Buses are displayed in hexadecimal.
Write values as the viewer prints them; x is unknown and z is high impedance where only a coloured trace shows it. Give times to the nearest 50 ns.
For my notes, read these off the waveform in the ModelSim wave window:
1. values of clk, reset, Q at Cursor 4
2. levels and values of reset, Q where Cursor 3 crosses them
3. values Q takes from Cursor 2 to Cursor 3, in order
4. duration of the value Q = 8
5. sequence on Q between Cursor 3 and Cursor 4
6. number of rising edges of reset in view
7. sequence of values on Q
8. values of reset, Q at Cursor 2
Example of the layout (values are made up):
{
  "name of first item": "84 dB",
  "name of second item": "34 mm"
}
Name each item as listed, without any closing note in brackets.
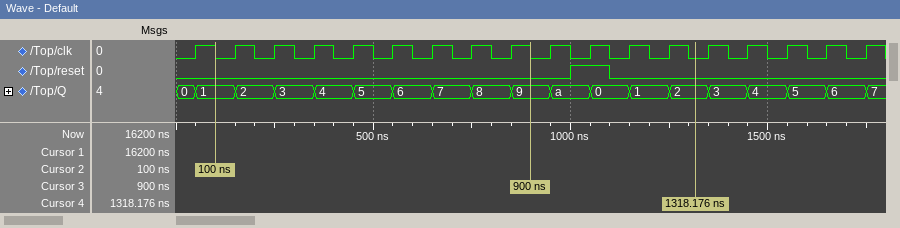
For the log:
{
  "values of clk, reset, Q at Cursor 4": "clk=0, reset=0, Q=2",
  "levels and values of reset, Q where Cursor 3 crosses them": "reset=0, Q=9",
  "values Q takes from Cursor 2 to Cursor 3, in order": "1, 2, 3, 4, 5, 6, 7, 8, 9",
  "duration of the value Q = 8": "100 ns",
  "sequence on Q between Cursor 3 and Cursor 4": "9, a, 0, 1, 2",
  "number of rising edges of reset in view": "1",
  "sequence of values on Q": "0, 1, 2, 3, 4, 5, 6, 7, 8, 9, a, 0, 1, 2, 3, 4, 5, 6, 7",
  "values of reset, Q at Cursor 2": "reset=0, Q=1"
}
